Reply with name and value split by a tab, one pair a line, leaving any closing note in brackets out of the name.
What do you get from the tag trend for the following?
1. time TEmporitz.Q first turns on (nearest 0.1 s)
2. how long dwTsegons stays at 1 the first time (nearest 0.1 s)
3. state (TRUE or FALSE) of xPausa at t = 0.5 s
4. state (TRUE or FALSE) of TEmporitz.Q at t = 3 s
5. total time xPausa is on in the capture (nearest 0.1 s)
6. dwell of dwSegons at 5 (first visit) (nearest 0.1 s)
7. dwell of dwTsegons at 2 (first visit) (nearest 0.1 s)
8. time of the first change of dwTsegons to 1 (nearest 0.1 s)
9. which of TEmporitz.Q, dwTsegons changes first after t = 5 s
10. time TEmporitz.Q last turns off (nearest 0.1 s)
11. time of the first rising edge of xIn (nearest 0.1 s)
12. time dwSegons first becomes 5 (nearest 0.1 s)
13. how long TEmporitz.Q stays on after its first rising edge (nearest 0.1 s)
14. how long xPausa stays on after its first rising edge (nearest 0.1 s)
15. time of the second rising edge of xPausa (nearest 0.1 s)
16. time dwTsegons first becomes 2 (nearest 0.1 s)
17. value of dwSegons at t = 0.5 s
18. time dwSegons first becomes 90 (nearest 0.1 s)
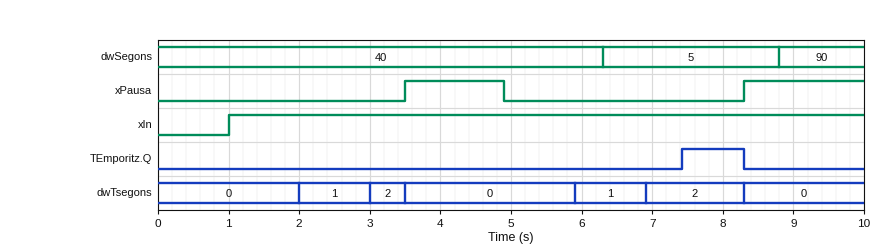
time TEmporitz.Q first turns on	7.4 s
how long dwTsegons stays at 1 the first time	1.0 s
state (TRUE or FALSE) of xPausa at t = 0.5 s	FALSE
state (TRUE or FALSE) of TEmporitz.Q at t = 3 s	FALSE
total time xPausa is on in the capture	3.1 s
dwell of dwSegons at 5 (first visit)	2.5 s
dwell of dwTsegons at 2 (first visit)	0.5 s
time of the first change of dwTsegons to 1	2.0 s
which of TEmporitz.Q, dwTsegons changes first after t = 5 s	dwTsegons
time TEmporitz.Q last turns off	8.3 s
time of the first rising edge of xIn	1.0 s
time dwSegons first becomes 5	6.3 s
how long TEmporitz.Q stays on after its first rising edge	0.9 s
how long xPausa stays on after its first rising edge	1.4 s
time of the second rising edge of xPausa	8.3 s
time dwTsegons first becomes 2	3.0 s
value of dwSegons at t = 0.5 s	40
time dwSegons first becomes 90	8.8 s
